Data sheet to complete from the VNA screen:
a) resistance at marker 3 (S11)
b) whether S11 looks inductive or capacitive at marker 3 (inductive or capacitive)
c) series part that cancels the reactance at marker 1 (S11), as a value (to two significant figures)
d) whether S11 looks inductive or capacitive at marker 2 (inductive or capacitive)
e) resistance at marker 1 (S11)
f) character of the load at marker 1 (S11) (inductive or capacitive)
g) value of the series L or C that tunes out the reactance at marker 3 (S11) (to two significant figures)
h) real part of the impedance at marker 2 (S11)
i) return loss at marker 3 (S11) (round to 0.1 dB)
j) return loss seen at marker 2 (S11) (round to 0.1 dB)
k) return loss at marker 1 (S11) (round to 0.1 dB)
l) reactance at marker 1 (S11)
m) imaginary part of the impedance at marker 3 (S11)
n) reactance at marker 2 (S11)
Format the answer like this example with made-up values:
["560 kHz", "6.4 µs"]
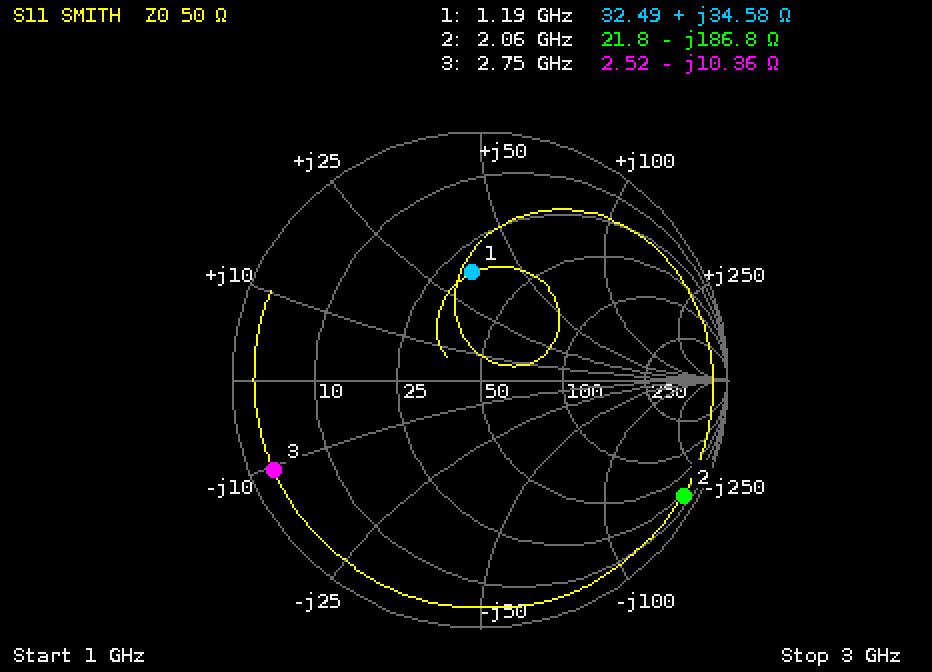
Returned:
["2.52 Ω", "capacitive", "3.9 pF", "capacitive", "32.49 Ω", "inductive", "600 pH", "21.8 Ω", "0.8 dB", "0.5 dB", "7.3 dB", "+34.58 Ω", "-10.36 Ω", "-186.8 Ω"]
